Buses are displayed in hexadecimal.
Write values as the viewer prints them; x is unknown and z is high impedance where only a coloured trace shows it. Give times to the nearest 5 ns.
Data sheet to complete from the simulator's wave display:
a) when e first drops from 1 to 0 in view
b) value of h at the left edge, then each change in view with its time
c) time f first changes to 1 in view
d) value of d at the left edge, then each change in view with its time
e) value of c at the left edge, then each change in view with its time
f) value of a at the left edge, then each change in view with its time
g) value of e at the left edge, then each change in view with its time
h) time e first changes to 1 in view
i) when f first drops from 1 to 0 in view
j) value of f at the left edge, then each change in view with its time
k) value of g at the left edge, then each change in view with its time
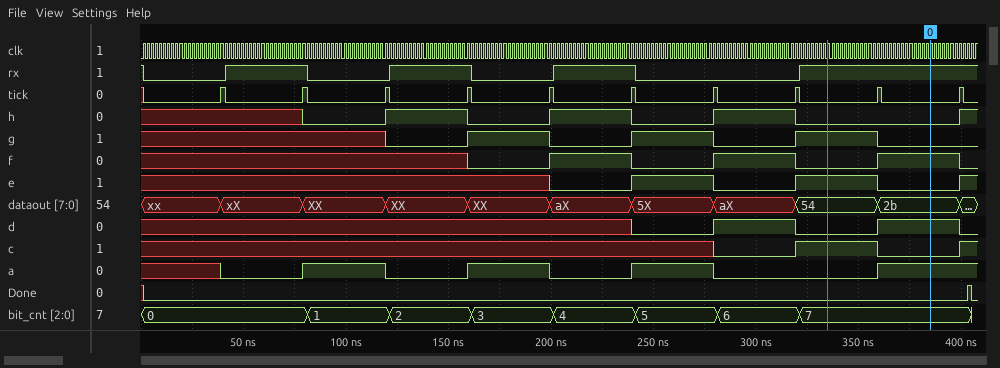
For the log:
280 ns
x, 0 at 80 ns, 1 at 120 ns, 0 at 160 ns, 1 at 200 ns, 0 at 240 ns, 1 at 280 ns, 0 at 320 ns, 1 at 400 ns
200 ns
x, 0 at 240 ns, 1 at 280 ns, 0 at 320 ns, 1 at 360 ns, 0 at 400 ns
x, 0 at 280 ns, 1 at 320 ns, 0 at 360 ns, 1 at 400 ns
x, 0 at 40 ns, 1 at 80 ns, 0 at 120 ns, 1 at 160 ns, 0 at 200 ns, 1 at 240 ns, 0 at 280 ns, 1 at 360 ns
x, 0 at 200 ns, 1 at 240 ns, 0 at 280 ns, 1 at 320 ns, 0 at 360 ns, 1 at 400 ns
240 ns
240 ns
x, 0 at 160 ns, 1 at 200 ns, 0 at 240 ns, 1 at 280 ns, 0 at 320 ns, 1 at 360 ns, 0 at 400 ns
x, 0 at 120 ns, 1 at 160 ns, 0 at 200 ns, 1 at 240 ns, 0 at 280 ns, 1 at 320 ns, 0 at 360 ns
